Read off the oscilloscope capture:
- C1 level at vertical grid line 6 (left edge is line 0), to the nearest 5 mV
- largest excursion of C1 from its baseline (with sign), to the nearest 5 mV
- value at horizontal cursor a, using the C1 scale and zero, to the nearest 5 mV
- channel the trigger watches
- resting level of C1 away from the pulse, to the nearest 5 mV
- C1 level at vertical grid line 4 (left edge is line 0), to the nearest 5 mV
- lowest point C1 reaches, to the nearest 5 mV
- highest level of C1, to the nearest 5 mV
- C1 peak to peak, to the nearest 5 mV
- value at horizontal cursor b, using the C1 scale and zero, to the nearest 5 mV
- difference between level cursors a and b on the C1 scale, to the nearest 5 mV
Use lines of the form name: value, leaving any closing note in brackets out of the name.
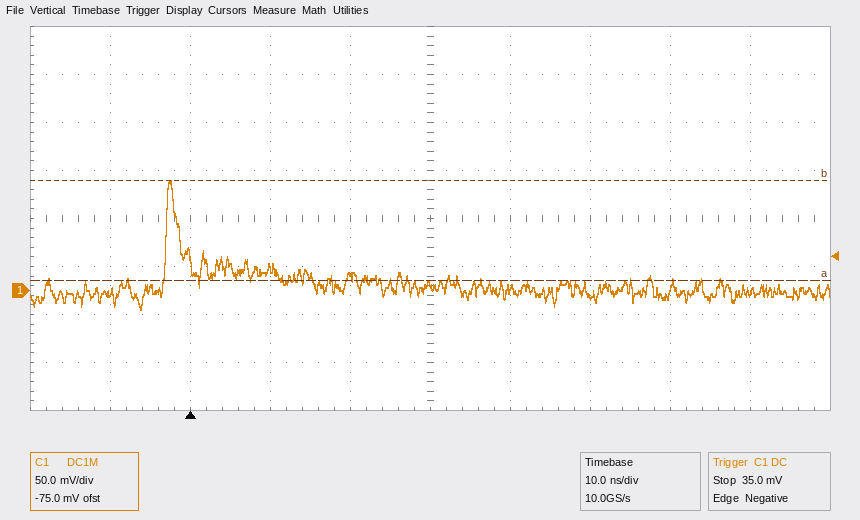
C1 level at vertical grid line 6 (left edge is line 0), to the nearest 5 mV: 0 mV
largest excursion of C1 from its baseline (with sign), to the nearest 5 mV: +115 mV
value at horizontal cursor a, using the C1 scale and zero, to the nearest 5 mV: 10 mV
channel the trigger watches: C1
resting level of C1 away from the pulse, to the nearest 5 mV: 0 mV
C1 level at vertical grid line 4 (left edge is line 0), to the nearest 5 mV: 15 mV
lowest point C1 reaches, to the nearest 5 mV: -20 mV
highest level of C1, to the nearest 5 mV: 115 mV
C1 peak to peak, to the nearest 5 mV: 135 mV
value at horizontal cursor b, using the C1 scale and zero, to the nearest 5 mV: 115 mV
difference between level cursors a and b on the C1 scale, to the nearest 5 mV: 105 mV
